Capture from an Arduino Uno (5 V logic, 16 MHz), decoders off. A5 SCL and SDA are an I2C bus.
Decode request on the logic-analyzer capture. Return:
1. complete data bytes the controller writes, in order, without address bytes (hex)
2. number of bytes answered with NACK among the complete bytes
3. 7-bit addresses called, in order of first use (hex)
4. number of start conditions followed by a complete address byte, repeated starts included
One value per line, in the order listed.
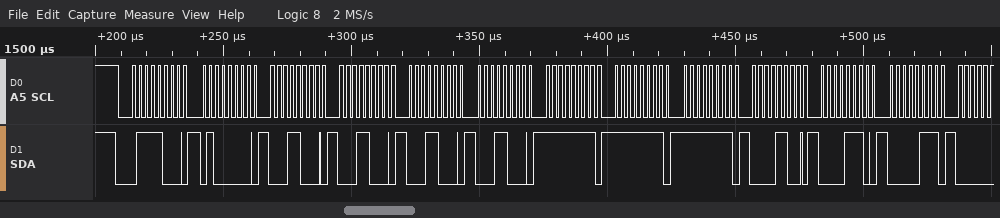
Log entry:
40 18 18 18 18 FF FF FF 0C 0E 07
0
0x3C
1
